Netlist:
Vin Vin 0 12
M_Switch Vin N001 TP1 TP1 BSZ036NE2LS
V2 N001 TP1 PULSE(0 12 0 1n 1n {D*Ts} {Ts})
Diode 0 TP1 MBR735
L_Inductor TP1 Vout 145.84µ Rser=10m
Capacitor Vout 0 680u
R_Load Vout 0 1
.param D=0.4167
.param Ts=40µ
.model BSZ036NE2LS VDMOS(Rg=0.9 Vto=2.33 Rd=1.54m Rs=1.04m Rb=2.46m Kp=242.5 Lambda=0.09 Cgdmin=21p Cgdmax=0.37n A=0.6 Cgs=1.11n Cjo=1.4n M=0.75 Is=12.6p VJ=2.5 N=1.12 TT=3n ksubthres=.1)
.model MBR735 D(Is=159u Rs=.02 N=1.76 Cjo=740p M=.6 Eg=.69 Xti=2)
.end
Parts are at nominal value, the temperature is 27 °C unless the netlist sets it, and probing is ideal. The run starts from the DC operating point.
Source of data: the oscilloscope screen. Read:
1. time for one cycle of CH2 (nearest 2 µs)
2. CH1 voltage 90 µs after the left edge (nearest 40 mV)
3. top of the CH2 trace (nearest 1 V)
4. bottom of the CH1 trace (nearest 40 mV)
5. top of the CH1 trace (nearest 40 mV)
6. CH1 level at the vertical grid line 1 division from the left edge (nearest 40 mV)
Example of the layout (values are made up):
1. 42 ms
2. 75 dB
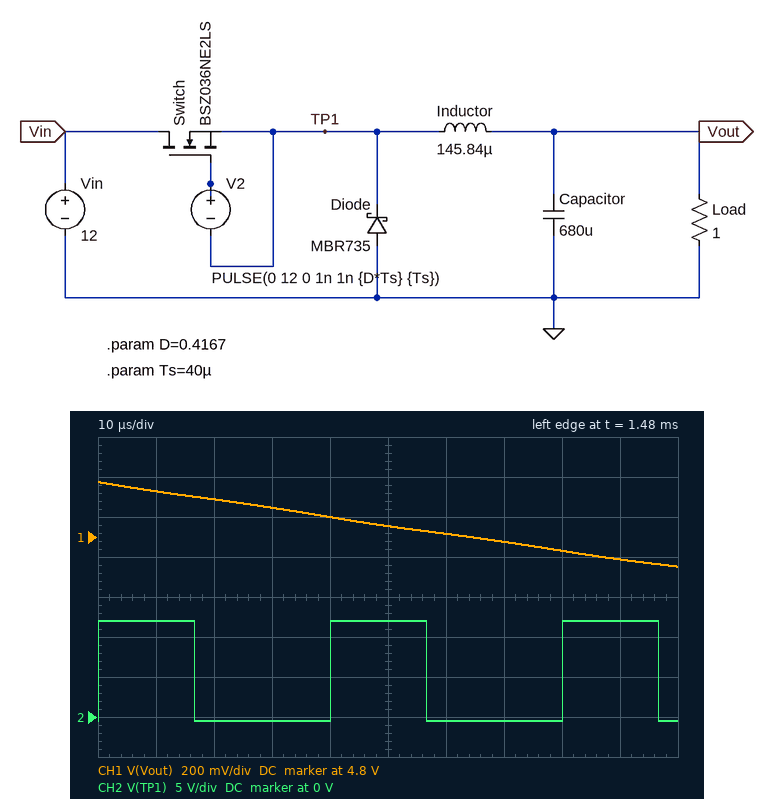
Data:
1. 40 µs
2. 4.68 V
3. 12 V
4. 4.64 V
5. 5.08 V
6. 5.04 V
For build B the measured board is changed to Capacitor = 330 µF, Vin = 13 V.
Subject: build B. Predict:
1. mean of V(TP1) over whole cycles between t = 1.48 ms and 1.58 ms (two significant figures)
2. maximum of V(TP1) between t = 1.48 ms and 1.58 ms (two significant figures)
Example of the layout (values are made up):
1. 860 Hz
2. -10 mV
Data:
1. 5.1 V
2. 13 V
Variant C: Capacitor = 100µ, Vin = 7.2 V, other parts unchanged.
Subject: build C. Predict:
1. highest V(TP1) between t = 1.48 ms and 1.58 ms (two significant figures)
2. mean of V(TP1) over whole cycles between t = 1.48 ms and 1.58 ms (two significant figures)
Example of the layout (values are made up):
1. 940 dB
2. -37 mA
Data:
1. 7.2 V
2. 2.7 V
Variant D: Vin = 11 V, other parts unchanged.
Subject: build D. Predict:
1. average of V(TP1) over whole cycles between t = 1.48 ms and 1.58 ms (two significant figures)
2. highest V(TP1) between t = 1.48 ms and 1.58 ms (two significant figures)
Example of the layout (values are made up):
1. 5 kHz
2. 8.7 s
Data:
1. 4.3 V
2. 11 V
